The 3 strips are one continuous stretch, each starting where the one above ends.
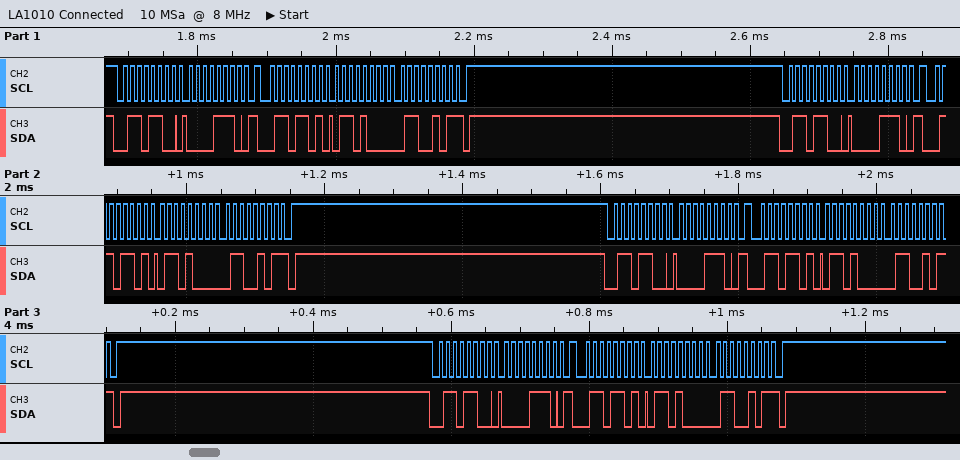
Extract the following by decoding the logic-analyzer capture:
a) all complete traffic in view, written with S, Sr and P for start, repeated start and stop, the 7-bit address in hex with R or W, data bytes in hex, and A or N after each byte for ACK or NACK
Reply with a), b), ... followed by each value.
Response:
a) S 36W A 0E A Sr 36R A 68 A 65 N P S 36W A 0E A Sr 36R A 68 A 65 N P S 36W A 0E A Sr 36R A 68 A 65 N P S 36W A 0E A Sr 36R A 68 A 65 N P
